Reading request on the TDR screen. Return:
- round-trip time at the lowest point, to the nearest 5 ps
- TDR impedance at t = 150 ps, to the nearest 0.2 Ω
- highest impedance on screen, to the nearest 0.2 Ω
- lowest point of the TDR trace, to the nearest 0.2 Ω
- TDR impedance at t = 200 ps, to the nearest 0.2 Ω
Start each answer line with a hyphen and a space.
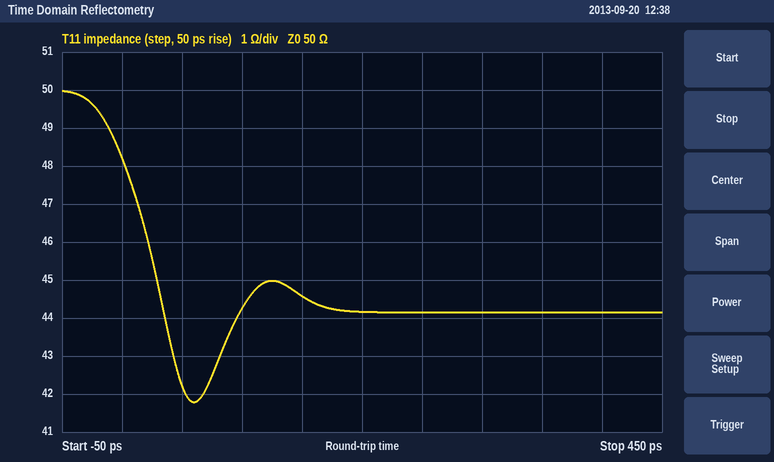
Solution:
- 60 ps
- 44.6 Ω
- 50.0 Ω
- 41.8 Ω
- 44.2 Ω
